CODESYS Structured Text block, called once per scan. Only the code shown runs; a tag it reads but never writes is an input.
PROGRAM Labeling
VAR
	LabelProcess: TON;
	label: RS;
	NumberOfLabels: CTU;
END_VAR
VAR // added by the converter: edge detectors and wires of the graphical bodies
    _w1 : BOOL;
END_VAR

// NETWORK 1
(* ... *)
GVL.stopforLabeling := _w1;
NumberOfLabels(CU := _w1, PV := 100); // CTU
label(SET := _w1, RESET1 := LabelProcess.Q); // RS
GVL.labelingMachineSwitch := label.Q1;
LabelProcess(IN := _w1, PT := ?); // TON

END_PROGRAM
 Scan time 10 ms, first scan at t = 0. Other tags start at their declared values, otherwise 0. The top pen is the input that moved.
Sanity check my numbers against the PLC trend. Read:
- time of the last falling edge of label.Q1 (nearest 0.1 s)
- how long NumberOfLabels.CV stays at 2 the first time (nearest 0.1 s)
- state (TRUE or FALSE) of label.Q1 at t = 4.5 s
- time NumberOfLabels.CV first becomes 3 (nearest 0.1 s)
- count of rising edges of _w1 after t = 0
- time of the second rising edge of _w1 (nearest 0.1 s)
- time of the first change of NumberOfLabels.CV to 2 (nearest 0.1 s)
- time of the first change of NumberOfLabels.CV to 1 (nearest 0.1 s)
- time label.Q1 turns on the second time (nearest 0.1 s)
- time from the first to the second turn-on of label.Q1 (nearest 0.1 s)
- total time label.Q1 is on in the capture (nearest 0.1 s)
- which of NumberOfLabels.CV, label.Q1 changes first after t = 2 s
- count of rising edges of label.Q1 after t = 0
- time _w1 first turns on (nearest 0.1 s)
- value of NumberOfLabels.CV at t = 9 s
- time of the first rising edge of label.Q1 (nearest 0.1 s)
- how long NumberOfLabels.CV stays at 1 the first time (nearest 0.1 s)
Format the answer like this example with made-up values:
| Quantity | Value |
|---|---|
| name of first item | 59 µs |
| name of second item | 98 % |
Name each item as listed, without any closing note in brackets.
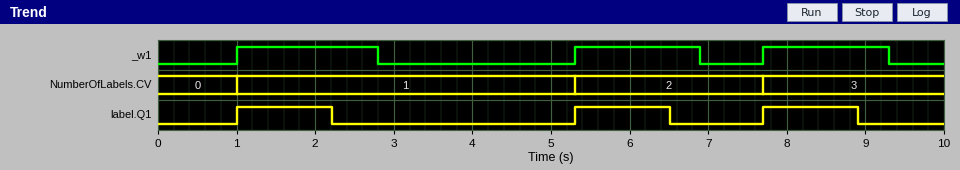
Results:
| Quantity | Value |
|---|---|
| time of the last falling edge of label.Q1 | 8.9 s |
| how long NumberOfLabels.CV stays at 2 the first time | 2.4 s |
| state (TRUE or FALSE) of label.Q1 at t = 4.5 s | FALSE |
| time NumberOfLabels.CV first becomes 3 | 7.7 s |
| count of rising edges of _w1 after t = 0 | 3 |
| time of the second rising edge of _w1 | 5.3 s |
| time of the first change of NumberOfLabels.CV to 2 | 5.3 s |
| time of the first change of NumberOfLabels.CV to 1 | 1.0 s |
| time label.Q1 turns on the second time | 5.3 s |
| time from the first to the second turn-on of label.Q1 | 4.3 s |
| total time label.Q1 is on in the capture | 3.6 s |
| which of NumberOfLabels.CV, label.Q1 changes first after t = 2 s | label.Q1 |
| count of rising edges of label.Q1 after t = 0 | 3 |
| time _w1 first turns on | 1.0 s |
| value of NumberOfLabels.CV at t = 9 s | 3 |
| time of the first rising edge of label.Q1 | 1.0 s |
| how long NumberOfLabels.CV stays at 1 the first time | 4.3 s |
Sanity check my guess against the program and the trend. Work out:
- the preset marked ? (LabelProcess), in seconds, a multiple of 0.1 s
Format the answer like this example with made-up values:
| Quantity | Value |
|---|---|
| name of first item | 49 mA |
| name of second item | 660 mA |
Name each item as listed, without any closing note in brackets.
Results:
| Quantity | Value |
|---|---|
| the preset marked ? (LabelProcess), in seconds, a multiple of 0.1 s | 1.2 s |
